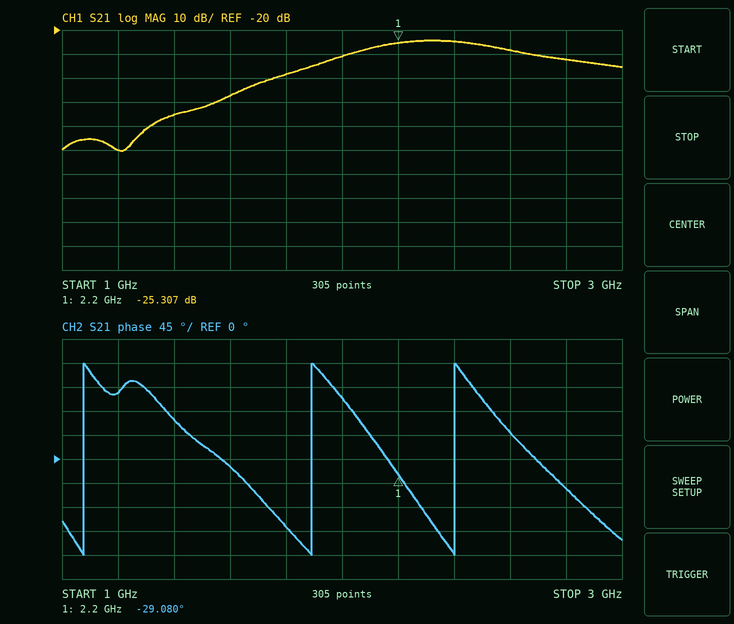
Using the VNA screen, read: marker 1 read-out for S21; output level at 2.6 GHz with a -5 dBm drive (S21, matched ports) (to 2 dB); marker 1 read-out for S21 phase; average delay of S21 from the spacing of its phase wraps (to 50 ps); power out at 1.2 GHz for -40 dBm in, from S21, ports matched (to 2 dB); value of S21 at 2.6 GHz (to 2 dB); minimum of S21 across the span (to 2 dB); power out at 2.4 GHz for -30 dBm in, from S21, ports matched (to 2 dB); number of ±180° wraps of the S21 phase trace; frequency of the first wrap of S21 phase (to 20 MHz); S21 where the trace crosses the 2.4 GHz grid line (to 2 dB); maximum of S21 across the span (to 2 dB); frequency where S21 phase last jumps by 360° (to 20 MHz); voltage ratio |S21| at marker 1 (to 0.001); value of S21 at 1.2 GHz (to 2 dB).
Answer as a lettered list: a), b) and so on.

a) -25.307 dB
b) -34 dBm
c) -29.080°
d) 1.50 ns
e) -110 dBm
f) -28 dB
g) -70 dB
h) -54 dBm
i) 3
j) 1.08 GHz
k) -24 dB
l) -24 dB
m) 2.40 GHz
n) 0.054
o) -70 dB
